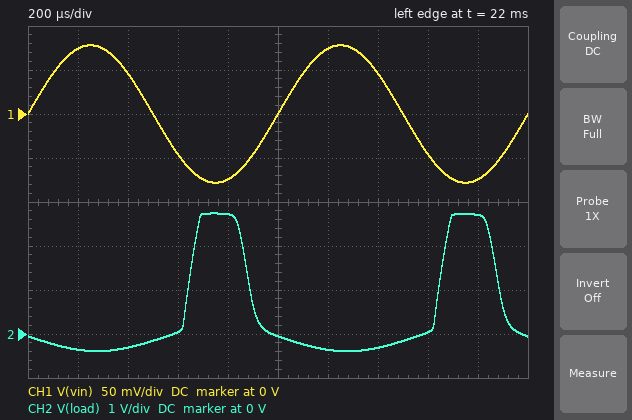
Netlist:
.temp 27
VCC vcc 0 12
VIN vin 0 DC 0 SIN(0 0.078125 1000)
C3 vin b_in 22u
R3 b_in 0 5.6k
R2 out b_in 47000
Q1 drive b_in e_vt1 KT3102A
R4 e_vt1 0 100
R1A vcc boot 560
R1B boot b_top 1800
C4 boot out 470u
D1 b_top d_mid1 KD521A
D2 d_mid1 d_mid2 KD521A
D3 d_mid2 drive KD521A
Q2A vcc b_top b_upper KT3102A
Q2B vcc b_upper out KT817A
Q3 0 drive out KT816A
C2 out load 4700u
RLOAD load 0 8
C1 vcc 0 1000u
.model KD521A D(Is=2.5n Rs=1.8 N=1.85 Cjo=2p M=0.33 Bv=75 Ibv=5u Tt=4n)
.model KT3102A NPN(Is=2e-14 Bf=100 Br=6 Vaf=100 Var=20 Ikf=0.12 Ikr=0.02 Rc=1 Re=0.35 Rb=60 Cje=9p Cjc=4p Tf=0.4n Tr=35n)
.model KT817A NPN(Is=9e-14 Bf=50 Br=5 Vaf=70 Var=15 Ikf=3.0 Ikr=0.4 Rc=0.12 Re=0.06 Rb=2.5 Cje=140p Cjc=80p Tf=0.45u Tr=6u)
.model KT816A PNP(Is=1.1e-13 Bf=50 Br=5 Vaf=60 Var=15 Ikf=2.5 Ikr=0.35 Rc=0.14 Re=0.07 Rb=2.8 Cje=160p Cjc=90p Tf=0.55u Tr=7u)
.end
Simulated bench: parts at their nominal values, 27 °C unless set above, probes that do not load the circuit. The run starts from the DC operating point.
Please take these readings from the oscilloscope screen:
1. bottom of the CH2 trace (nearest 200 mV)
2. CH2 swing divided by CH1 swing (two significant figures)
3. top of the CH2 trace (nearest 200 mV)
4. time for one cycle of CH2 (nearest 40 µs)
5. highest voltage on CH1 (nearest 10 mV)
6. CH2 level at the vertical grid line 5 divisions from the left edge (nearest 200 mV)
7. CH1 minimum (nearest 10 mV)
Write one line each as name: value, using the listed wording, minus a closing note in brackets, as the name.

bottom of the CH2 trace: -400 mV
CH2 swing divided by CH1 swing: 20
top of the CH2 trace: 2.8 V
time for one cycle of CH2: 1.00 ms
highest voltage on CH1: 80 mV
CH2 level at the vertical grid line 5 divisions from the left edge: 0 V
CH1 minimum: -80 mV
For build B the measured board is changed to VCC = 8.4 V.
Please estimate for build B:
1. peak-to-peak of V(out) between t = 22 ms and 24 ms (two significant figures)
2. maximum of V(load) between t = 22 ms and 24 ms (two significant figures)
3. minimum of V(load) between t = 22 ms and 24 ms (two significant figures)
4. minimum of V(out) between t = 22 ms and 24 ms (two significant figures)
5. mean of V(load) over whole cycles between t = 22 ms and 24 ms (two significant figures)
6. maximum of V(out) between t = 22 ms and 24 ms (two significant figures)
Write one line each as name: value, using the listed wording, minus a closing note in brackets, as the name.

peak-to-peak of V(out) between t = 22 ms and 24 ms: 1.3 V
maximum of V(load) between t = 22 ms and 24 ms: 1.1 V
minimum of V(load) between t = 22 ms and 24 ms: -250 mV
minimum of V(out) between t = 22 ms and 24 ms: 6.3 V
mean of V(load) over whole cycles between t = 22 ms and 24 ms: 270 mV
maximum of V(out) between t = 22 ms and 24 ms: 7.6 V
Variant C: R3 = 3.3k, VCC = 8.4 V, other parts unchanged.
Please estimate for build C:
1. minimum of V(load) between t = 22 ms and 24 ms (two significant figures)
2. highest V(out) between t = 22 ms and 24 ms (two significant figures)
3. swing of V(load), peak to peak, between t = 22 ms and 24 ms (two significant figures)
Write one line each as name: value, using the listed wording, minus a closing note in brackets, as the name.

minimum of V(load) between t = 22 ms and 24 ms: -1.2 mV
highest V(out) between t = 22 ms and 24 ms: 7.4 V
swing of V(load), peak to peak, between t = 22 ms and 24 ms: 1.3 mV
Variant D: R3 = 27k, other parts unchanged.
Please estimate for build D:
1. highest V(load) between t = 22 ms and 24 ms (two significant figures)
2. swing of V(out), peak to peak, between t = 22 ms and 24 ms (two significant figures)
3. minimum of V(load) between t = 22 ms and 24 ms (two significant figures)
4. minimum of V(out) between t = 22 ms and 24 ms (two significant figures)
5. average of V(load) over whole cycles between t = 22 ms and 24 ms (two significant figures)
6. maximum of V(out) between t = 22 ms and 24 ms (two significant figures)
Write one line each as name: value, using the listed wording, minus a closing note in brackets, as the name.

highest V(load) between t = 22 ms and 24 ms: 770 mV
swing of V(out), peak to peak, between t = 22 ms and 24 ms: 1.1 V
minimum of V(load) between t = 22 ms and 24 ms: -370 mV
minimum of V(out) between t = 22 ms and 24 ms: 4.1 V
average of V(load) over whole cycles between t = 22 ms and 24 ms: 66 mV
maximum of V(out) between t = 22 ms and 24 ms: 5.2 V
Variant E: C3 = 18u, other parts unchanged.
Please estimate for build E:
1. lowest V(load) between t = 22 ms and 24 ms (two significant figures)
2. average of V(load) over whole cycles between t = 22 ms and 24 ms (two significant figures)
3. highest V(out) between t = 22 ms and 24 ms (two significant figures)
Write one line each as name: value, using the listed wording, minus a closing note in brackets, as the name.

lowest V(load) between t = 22 ms and 24 ms: -400 mV
average of V(load) over whole cycles between t = 22 ms and 24 ms: 430 mV
highest V(out) between t = 22 ms and 24 ms: 11 V
